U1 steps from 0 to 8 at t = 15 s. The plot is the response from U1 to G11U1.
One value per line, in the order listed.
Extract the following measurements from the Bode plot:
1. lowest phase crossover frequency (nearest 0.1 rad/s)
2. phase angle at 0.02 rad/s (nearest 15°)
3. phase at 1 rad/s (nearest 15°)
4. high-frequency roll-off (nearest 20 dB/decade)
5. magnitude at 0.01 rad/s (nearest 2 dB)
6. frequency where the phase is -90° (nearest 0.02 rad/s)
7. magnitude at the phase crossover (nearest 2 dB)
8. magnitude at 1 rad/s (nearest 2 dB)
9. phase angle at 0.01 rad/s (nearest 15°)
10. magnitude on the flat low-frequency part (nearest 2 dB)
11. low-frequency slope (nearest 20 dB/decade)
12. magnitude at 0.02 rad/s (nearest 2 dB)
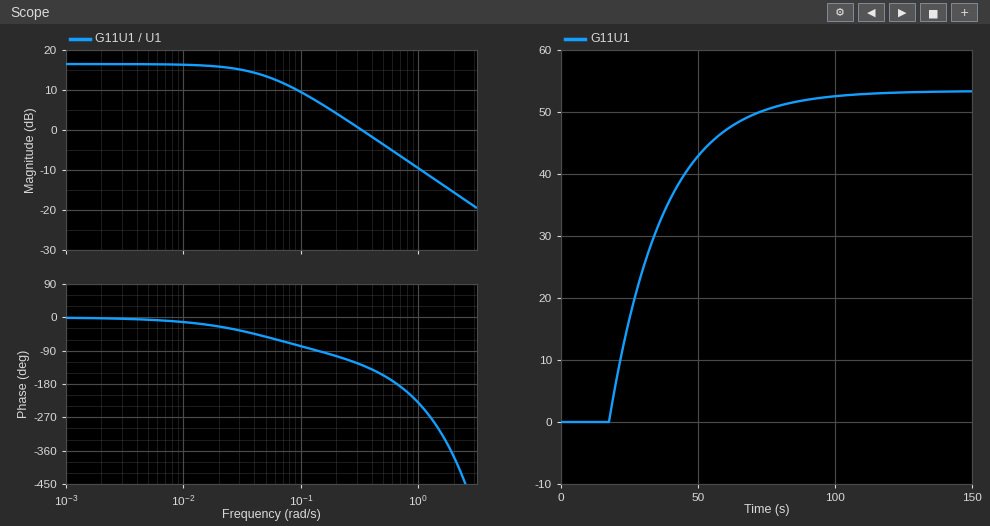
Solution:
0.7 rad/s
-30°
-225°
-20 dB/decade
16 dB
0.14 rad/s
-6 dB
-10 dB
-15°
16 dB
0 dB/decade
16 dB
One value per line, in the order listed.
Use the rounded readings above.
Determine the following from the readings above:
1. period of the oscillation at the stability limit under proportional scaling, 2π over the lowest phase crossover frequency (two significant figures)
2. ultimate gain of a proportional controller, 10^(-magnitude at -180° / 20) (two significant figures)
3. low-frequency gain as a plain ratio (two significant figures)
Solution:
9.0 s
2.0
6.3
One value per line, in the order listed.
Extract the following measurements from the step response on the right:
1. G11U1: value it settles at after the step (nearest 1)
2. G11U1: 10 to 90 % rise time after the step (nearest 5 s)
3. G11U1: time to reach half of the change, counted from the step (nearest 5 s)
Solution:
53
45 s
15 s
